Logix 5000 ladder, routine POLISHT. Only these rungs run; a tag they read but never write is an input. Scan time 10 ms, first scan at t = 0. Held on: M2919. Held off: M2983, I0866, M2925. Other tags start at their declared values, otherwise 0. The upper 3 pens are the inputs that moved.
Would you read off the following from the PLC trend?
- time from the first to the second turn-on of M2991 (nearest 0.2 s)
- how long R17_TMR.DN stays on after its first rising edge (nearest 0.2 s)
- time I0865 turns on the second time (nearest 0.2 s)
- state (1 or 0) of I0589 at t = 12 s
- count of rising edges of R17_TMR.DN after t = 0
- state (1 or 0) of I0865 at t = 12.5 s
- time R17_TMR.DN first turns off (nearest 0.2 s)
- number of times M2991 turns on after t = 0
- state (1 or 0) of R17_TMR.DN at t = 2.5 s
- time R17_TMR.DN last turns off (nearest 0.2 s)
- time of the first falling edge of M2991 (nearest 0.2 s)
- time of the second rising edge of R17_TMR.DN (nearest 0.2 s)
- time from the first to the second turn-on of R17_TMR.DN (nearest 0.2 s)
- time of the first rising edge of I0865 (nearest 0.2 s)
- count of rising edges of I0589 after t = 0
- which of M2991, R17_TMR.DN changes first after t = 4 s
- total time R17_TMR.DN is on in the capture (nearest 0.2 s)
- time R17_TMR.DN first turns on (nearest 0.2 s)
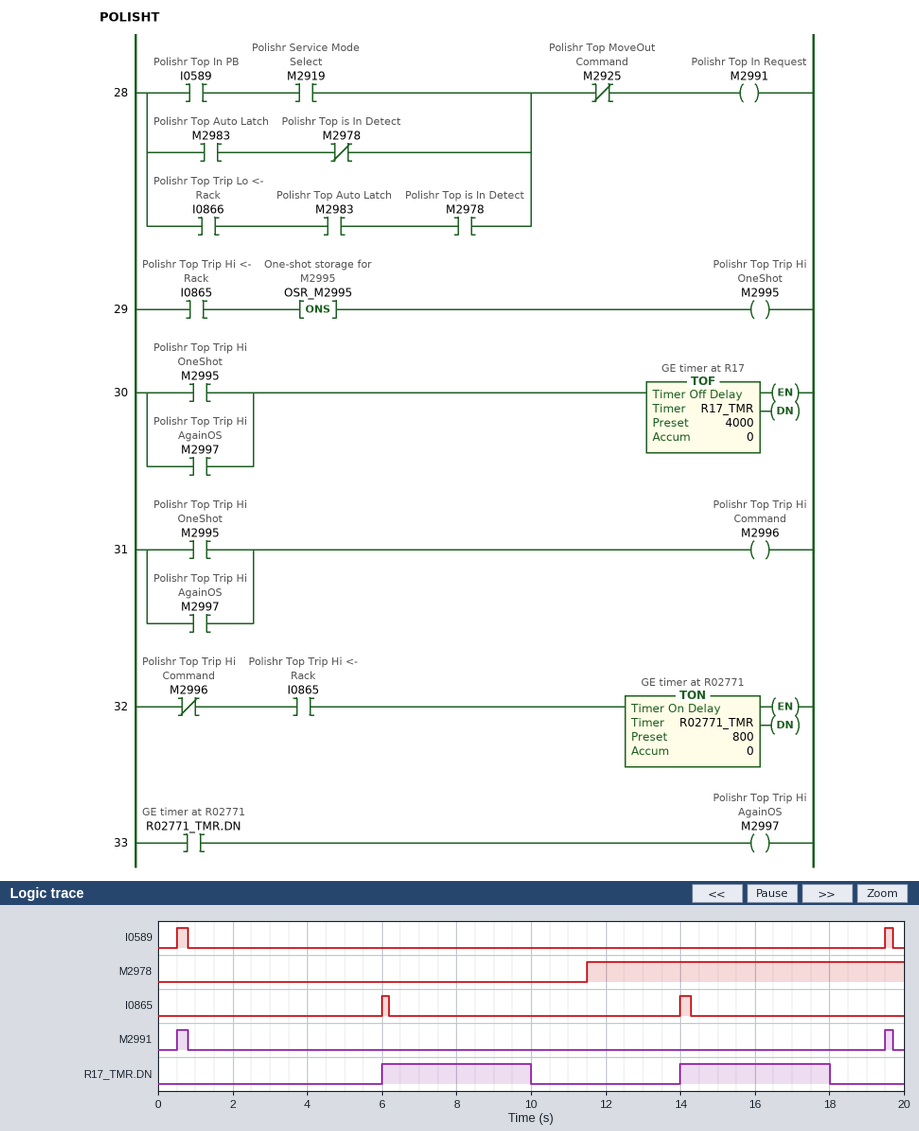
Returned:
19.0 s
4.0 s
14.0 s
0
2
0
10.0 s
2
0
18.0 s
0.8 s
14.0 s
8.0 s
6.0 s
2
R17_TMR.DN
8.0 s
6.0 s
